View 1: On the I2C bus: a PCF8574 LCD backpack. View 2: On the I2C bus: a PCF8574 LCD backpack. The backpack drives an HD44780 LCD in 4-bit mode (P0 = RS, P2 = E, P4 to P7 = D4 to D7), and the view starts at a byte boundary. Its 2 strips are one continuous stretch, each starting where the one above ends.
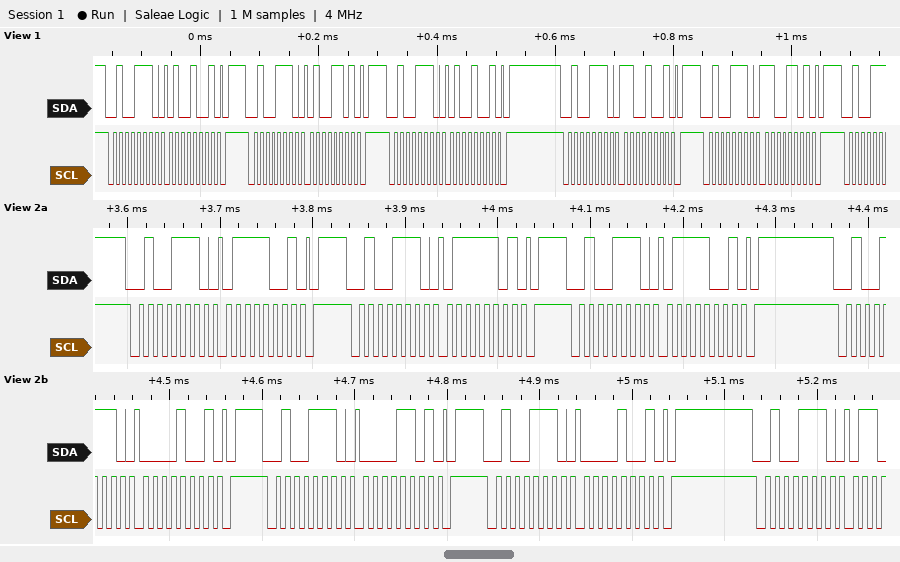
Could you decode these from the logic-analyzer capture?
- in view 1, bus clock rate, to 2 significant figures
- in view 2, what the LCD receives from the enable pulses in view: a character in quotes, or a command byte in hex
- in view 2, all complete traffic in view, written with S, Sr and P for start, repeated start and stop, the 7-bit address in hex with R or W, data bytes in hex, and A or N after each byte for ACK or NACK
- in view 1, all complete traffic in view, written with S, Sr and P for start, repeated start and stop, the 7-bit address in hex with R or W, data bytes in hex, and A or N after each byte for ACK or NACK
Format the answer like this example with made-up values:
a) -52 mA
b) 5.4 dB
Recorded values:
a) 100 kHz
b) 'p'
c) S 27W A 79 A P S 27W A 7D A P S 27W A 79 A P S 27W A 09 A P S 27W A 0D A P S 27W A 09 A P S 27W A
d) S 27W A 49 A P S 27W A 4D A P S 27W A 49 A P S 27W A C9 A P S 27W A CD A P
